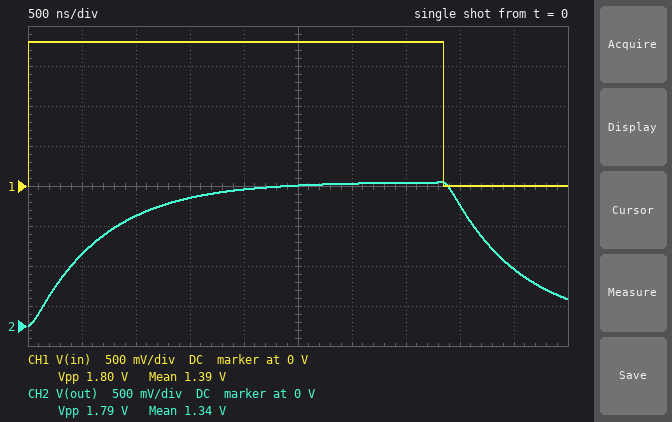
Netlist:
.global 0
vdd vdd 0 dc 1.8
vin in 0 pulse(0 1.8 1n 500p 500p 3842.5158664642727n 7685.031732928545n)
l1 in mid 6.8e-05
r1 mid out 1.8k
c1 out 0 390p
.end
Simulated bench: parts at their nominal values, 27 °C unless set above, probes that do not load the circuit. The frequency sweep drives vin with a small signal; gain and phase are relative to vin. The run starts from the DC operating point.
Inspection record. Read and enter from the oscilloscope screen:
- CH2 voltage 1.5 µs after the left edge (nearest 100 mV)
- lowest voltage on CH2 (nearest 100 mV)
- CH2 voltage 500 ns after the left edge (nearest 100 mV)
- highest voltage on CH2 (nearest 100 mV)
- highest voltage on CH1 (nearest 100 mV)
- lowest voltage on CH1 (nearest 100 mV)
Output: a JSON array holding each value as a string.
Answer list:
["1.6 V", "0 V", "900 mV", "1.8 V", "1.8 V", "0 V"]
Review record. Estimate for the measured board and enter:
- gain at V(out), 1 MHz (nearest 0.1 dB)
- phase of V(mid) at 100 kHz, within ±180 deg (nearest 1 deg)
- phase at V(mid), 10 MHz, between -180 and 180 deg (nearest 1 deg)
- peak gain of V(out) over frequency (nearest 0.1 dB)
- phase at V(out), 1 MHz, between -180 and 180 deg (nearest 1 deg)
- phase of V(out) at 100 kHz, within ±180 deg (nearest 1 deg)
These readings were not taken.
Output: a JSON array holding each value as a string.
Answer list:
["-12.9 dB", "0 deg", "-68 deg", "0 dB", "-91 deg", "-24 deg"]
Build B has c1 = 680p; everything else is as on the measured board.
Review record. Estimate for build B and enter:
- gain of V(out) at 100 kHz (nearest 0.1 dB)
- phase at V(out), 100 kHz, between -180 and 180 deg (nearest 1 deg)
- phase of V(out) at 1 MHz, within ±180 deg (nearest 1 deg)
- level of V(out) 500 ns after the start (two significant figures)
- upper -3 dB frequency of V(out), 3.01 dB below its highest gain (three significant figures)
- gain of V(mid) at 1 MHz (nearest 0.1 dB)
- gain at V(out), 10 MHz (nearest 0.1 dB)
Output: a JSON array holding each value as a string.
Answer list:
["-1.9 dB", "-38 deg", "-96 deg", "580 mV", "134 kHz", "0 dB", "-45.9 dB"]
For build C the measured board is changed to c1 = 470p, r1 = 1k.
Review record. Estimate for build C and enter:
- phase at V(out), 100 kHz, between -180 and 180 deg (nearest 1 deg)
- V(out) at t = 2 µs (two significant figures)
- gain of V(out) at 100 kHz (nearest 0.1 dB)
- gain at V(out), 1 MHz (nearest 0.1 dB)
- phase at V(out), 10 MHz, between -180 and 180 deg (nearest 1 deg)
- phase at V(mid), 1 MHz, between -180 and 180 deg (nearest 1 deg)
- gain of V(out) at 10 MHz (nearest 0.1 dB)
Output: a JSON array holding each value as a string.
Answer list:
["-17 deg", "1.8 V", "-0.3 dB", "-9.4 dB", "-167 deg", "-24 deg", "-42.2 dB"]
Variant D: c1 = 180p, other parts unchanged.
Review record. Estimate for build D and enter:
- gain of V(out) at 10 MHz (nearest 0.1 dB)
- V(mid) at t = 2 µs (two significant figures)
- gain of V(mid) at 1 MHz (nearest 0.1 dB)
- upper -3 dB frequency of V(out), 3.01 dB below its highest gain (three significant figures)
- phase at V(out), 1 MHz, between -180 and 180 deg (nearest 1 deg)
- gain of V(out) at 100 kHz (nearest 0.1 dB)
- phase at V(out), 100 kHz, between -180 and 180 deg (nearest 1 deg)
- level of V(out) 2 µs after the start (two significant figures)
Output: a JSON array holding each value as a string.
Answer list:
["-34.2 dB", "1.8 V", "0.7 dB", "555 kHz", "-76 deg", "-0.1 dB", "-12 deg", "1.8 V"]
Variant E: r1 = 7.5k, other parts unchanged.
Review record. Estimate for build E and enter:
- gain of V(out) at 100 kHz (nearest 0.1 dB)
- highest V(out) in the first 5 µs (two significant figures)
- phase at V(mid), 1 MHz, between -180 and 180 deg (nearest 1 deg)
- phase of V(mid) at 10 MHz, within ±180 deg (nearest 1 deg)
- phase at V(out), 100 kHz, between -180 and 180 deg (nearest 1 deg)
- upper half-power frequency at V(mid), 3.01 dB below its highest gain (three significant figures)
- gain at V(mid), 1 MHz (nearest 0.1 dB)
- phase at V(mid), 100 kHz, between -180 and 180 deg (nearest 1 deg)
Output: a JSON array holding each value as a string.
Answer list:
["-6.4 dB", "1.3 V", "-3 deg", "-30 deg", "-62 deg", "17.5 MHz", "0 dB", "0 deg"]
